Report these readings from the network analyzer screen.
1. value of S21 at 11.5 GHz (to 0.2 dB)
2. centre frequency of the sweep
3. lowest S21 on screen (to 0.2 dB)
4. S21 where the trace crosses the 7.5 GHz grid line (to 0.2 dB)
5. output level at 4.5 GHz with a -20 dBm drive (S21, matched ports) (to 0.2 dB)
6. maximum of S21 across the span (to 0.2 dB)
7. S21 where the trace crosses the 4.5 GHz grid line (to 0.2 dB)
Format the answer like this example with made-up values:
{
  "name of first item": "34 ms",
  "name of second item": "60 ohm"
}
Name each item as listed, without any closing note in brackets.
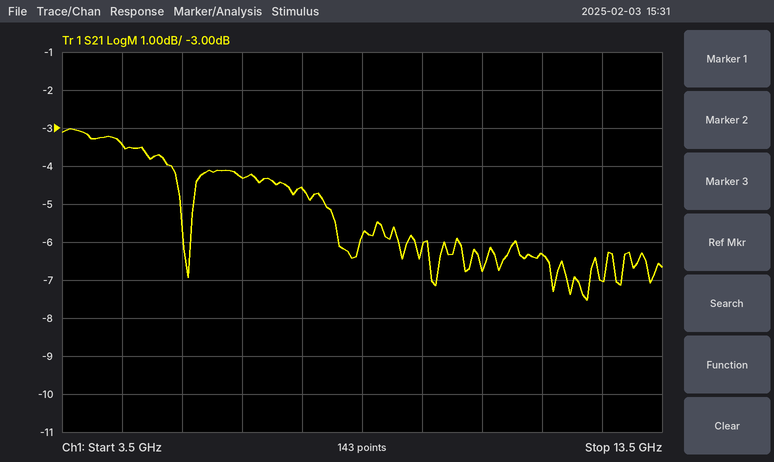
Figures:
{
  "value of S21 at 11.5 GHz": "-6.4 dB",
  "centre frequency of the sweep": "8.5 GHz",
  "lowest S21 on screen": "-7.6 dB",
  "S21 where the trace crosses the 7.5 GHz grid line": "-4.6 dB",
  "output level at 4.5 GHz with a -20 dBm drive (S21, matched ports)": "-23.4 dBm",
  "maximum of S21 across the span": "-3.0 dB",
  "S21 where the trace crosses the 4.5 GHz grid line": "-3.4 dB"
}
